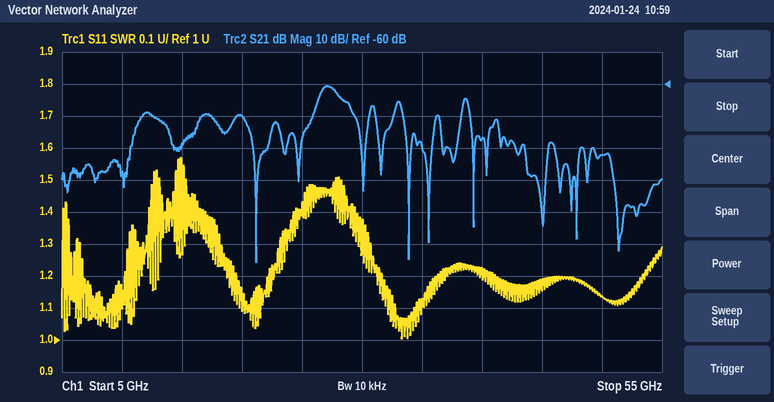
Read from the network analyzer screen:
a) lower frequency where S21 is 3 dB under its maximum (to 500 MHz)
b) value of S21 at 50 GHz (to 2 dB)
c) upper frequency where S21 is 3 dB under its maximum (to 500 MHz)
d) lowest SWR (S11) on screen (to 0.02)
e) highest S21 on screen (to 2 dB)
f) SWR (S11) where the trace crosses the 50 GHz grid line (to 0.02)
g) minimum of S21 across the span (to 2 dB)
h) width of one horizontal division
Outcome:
26.5 GHz
-82 dB
28.0 GHz
1.00
-60 dB
1.14
-116 dB
5 GHz
